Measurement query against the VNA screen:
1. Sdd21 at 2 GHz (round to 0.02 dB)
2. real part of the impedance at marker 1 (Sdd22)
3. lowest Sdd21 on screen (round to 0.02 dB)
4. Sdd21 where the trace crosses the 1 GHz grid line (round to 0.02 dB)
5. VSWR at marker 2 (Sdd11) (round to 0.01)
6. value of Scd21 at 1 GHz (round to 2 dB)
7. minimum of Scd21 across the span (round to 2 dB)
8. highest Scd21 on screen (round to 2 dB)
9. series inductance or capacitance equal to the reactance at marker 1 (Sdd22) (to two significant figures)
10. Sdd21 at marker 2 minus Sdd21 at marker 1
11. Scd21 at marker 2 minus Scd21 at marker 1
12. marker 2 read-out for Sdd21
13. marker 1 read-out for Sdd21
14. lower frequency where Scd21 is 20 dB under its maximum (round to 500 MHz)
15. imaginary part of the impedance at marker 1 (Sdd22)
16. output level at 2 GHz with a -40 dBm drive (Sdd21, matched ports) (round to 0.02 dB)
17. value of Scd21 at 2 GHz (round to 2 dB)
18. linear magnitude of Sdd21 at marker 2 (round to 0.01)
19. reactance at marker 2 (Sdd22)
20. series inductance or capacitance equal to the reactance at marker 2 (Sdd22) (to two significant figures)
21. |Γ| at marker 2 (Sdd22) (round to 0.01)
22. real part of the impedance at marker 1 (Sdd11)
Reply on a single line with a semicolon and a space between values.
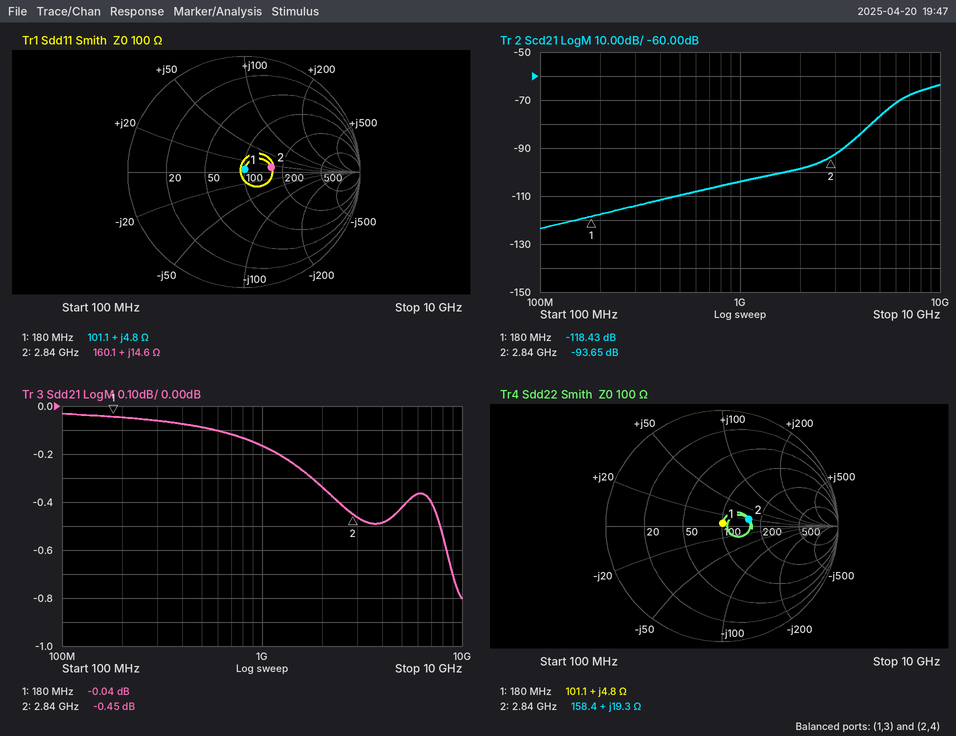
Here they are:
-0.34 dB; 101.1 Ω; -0.80 dB; -0.16 dB; 1.62; -104 dB; -124 dB; -64 dB; 4.2 nH; -0.41 dB; 24.78 dB; -0.45 dB; -0.04 dB; 4.0 GHz; +4.8 Ω; -40.34 dBm; -98 dB; 0.95; +19.3 Ω; 1.1 nH; 0.24; 101.1 Ω
